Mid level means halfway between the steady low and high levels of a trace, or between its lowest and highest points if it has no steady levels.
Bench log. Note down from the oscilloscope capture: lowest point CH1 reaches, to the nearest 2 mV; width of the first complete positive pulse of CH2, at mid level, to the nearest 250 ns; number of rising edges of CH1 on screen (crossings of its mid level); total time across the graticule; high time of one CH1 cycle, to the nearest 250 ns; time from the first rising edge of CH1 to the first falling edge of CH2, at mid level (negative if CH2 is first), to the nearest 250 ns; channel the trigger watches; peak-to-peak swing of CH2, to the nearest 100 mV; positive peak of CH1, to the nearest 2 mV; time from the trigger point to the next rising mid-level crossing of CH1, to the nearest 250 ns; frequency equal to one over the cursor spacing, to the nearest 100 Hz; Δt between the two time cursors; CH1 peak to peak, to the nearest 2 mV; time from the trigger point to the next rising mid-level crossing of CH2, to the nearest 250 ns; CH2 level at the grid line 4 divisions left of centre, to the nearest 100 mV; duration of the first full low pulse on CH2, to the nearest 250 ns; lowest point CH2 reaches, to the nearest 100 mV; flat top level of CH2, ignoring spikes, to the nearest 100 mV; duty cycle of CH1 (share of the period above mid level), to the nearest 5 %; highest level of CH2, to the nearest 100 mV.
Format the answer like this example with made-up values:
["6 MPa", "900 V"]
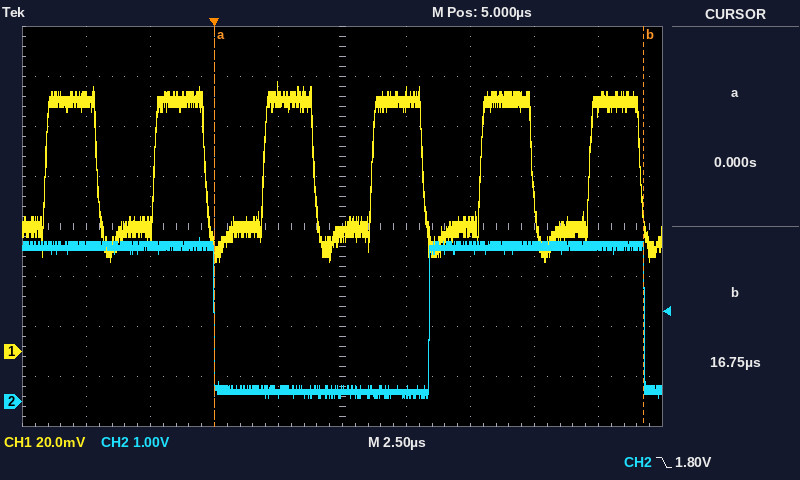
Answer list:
["36 mV", "8.50 µs", "6", "25 µs", "2.00 µs", "+6.50 µs", "CH2", "3.2 V", "108 mV", "2.00 µs", "59.7 kHz", "16.75 µs", "72 mV", "8.50 µs", "3.1 V", "8.50 µs", "100 mV", "3.1 V", "45 %", "3.3 V"]
